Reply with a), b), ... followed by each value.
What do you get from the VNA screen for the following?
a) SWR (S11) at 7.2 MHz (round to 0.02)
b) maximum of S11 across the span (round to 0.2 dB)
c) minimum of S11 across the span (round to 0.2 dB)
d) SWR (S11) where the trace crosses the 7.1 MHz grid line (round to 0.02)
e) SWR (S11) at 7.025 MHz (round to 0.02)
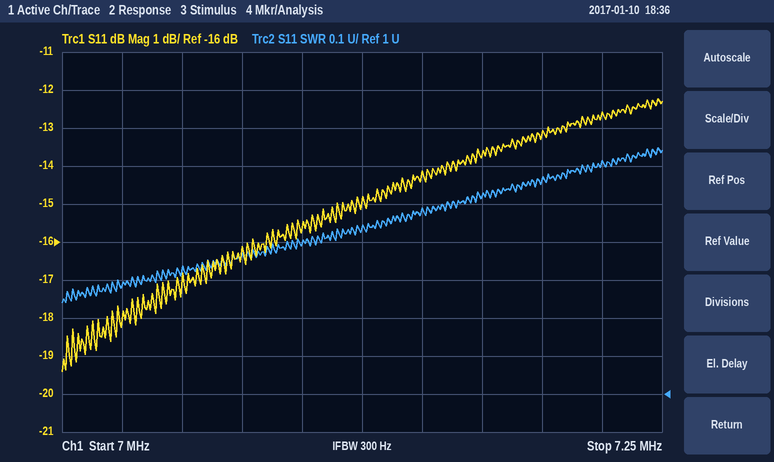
a) 1.56
b) -12.2 dB
c) -19.4 dB
d) 1.40
e) 1.28
